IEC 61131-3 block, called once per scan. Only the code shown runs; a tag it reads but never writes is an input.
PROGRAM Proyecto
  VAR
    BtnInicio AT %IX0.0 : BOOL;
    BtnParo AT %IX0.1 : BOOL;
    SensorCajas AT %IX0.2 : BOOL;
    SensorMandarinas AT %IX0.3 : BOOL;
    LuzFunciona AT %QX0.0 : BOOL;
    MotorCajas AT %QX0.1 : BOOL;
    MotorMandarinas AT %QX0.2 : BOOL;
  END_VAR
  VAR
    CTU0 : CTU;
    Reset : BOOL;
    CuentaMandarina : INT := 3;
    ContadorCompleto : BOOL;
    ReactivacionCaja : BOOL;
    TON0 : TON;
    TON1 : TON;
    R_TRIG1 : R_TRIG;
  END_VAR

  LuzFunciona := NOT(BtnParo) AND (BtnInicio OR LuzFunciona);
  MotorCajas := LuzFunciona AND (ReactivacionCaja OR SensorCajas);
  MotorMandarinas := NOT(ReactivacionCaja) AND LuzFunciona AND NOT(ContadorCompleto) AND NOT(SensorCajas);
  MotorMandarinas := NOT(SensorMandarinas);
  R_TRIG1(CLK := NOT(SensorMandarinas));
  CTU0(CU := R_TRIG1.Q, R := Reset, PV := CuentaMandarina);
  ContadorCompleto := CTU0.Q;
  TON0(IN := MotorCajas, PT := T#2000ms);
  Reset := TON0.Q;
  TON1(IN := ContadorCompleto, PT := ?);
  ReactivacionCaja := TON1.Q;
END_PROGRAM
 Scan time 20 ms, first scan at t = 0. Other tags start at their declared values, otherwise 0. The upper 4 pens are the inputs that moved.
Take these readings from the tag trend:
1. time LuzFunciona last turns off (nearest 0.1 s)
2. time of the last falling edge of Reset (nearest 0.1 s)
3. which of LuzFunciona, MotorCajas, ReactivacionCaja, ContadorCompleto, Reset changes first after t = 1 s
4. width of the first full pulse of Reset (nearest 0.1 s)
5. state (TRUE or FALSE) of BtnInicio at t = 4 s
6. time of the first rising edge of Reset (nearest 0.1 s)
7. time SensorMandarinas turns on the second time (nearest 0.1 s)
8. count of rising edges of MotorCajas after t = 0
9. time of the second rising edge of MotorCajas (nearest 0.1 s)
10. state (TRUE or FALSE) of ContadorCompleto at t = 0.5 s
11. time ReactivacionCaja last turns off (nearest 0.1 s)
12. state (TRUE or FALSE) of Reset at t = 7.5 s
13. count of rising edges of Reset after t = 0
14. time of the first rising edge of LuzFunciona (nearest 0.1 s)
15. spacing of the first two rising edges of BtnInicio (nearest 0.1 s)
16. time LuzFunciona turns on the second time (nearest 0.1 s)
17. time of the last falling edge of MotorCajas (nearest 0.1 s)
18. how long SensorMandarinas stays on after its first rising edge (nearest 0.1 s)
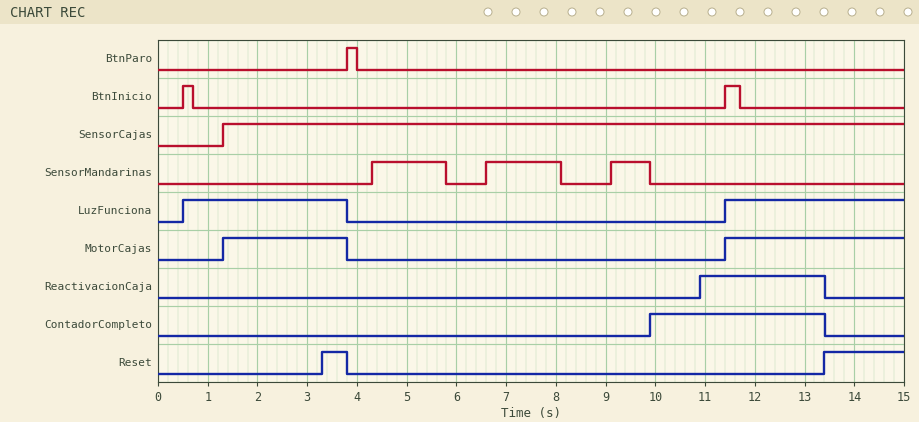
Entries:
3.8 s
3.8 s
MotorCajas
0.5 s
FALSE
3.3 s
6.6 s
2
11.4 s
FALSE
13.4 s
FALSE
2
0.5 s
10.9 s
11.4 s
3.8 s
1.5 s
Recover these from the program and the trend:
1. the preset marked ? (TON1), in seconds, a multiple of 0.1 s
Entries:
1.0 s
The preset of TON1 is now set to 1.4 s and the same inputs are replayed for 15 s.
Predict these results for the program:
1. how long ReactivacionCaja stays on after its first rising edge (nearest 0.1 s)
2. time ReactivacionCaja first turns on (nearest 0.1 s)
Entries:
2.1 s
11.3 s
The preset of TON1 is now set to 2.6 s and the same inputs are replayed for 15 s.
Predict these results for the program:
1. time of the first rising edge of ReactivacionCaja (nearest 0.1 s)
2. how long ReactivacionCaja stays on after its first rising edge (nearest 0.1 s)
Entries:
12.5 s
0.9 s
